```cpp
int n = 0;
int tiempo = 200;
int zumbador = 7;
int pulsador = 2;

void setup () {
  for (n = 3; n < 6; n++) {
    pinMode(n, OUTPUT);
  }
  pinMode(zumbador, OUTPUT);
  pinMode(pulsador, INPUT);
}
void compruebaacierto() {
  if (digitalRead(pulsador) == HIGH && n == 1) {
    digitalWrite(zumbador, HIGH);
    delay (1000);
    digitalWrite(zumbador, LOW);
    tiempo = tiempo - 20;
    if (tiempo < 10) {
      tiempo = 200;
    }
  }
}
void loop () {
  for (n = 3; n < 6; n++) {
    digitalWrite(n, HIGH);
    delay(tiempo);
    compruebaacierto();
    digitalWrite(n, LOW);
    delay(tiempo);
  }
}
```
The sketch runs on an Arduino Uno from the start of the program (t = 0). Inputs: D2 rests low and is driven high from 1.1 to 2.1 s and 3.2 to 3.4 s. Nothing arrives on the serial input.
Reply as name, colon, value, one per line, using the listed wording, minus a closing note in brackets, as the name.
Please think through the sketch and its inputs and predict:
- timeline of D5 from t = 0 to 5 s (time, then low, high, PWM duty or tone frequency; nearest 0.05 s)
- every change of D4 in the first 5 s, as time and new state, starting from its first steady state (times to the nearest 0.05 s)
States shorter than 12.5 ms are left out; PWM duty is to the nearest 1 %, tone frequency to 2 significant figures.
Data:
timeline of D5 from t = 0 to 5 s: 0 s low; 0.8 s high; 1 s low; 2 s high; 2.2 s low; 3.2 s high; 3.4 s low; 4.4 s high; 4.6 s low
every change of D4 in the first 5 s, as time and new state, starting from its first steady state: 0 s low; 0.4 s high; 0.6 s low; 1.6 s high; 1.8 s low; 2.8 s high; 3 s low; 4 s high; 4.2 s low
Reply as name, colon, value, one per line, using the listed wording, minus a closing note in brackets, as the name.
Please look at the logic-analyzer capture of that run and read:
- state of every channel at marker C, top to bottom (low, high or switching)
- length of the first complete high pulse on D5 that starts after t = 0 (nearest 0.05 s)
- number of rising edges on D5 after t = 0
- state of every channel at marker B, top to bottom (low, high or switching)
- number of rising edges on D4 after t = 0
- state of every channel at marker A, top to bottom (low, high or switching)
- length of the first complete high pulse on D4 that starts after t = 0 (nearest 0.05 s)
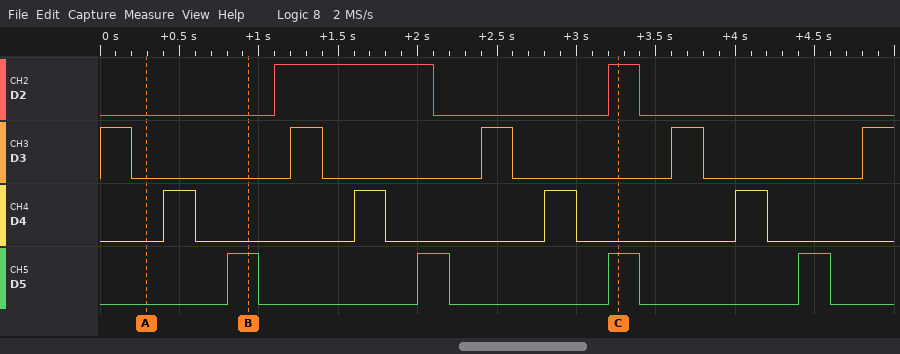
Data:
state of every channel at marker C, top to bottom: D2 high, D3 low, D4 low, D5 high
length of the first complete high pulse on D5 that starts after t = 0: 0.20 s
number of rising edges on D5 after t = 0: 4
state of every channel at marker B, top to bottom: D2 low, D3 low, D4 low, D5 high
number of rising edges on D4 after t = 0: 4
state of every channel at marker A, top to bottom: D2 low, D3 low, D4 low, D5 low
length of the first complete high pulse on D4 that starts after t = 0: 0.20 s
